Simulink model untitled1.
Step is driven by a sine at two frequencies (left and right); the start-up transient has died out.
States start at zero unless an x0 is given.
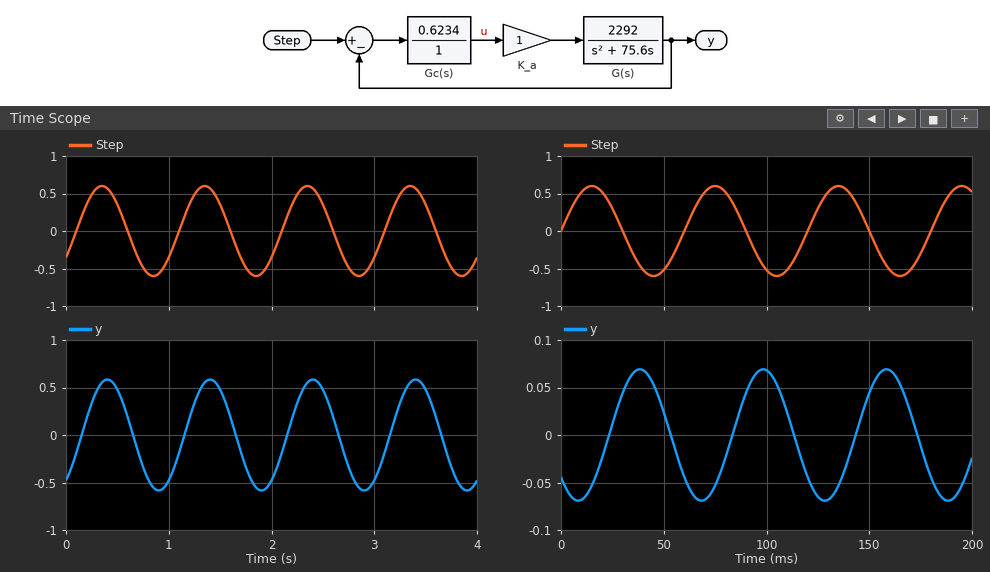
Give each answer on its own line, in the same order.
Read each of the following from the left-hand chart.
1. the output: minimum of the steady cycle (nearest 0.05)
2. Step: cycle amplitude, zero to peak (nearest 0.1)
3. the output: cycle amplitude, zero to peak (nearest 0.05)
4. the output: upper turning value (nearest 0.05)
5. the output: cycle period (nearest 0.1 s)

-0.60
0.6
0.60
0.60
1.0 s
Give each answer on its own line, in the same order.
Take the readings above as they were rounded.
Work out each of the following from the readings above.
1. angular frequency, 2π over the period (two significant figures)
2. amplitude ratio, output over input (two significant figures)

6.3 rad/s
1.0
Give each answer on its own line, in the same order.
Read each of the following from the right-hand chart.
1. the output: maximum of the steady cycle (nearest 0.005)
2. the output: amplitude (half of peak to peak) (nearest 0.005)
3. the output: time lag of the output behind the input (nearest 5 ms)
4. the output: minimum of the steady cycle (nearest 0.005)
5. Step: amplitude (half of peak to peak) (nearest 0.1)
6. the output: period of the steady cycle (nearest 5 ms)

0.070
0.070
25 ms
-0.070
0.6
60 ms
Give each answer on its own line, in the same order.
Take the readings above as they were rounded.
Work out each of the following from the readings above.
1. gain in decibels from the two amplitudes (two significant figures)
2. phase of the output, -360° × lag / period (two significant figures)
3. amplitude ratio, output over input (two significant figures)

-19 dB
-150°
0.12
